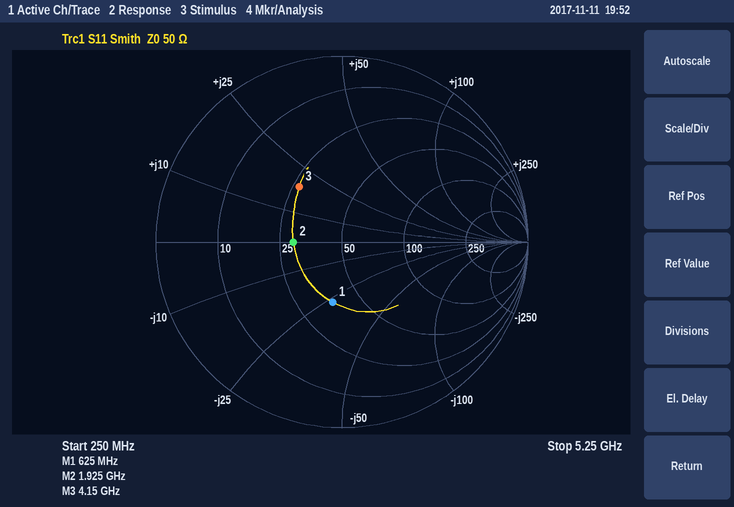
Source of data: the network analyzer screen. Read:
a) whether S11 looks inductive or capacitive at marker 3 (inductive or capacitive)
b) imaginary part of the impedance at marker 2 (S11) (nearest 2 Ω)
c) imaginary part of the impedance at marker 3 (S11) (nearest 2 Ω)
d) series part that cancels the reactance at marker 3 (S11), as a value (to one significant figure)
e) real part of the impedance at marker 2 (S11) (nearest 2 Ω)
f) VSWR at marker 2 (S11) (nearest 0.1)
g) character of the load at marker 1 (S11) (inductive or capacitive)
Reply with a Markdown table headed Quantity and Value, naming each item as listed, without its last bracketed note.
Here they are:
| Quantity | Value |
|---|---|
| whether S11 looks inductive or capacitive at marker 3 | inductive |
| imaginary part of the impedance at marker 2 (S11) | 0 Ω |
| imaginary part of the impedance at marker 3 (S11) | +18 Ω |
| series part that cancels the reactance at marker 3 (S11), as a value | 2 pF |
| real part of the impedance at marker 2 (S11) | 30 Ω |
| VSWR at marker 2 (S11) | 1.7 |
| character of the load at marker 1 (S11) | capacitive |
